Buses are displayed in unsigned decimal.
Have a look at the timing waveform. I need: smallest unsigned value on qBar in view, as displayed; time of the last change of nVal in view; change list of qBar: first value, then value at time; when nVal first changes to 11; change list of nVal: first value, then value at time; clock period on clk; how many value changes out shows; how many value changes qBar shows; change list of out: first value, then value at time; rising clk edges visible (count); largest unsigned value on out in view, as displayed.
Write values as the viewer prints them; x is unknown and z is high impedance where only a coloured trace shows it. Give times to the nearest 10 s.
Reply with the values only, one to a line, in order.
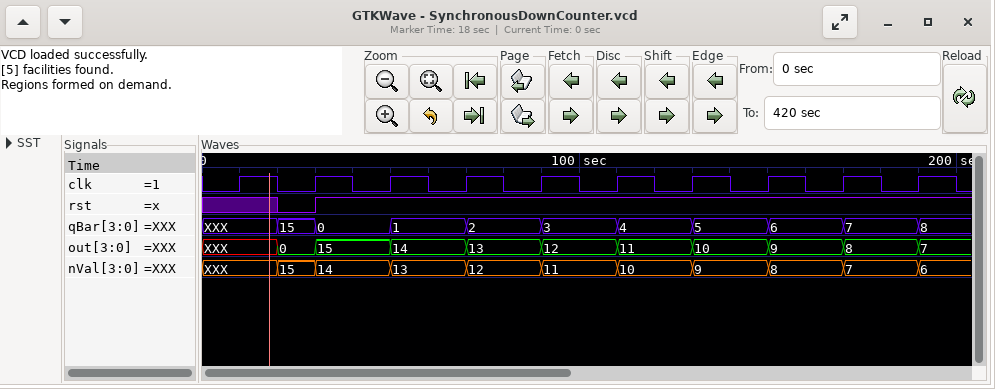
0
190 s
XXX, 15 at 20 s, 0 at 30 s, 1 at 50 s, 2 at 70 s, 3 at 90 s, 4 at 110 s, 5 at 130 s, 6 at 150 s, 7 at 170 s, 8 at 190 s
90 s
XXX, 15 at 20 s, 14 at 30 s, 13 at 50 s, 12 at 70 s, 11 at 90 s, 10 at 110 s, 9 at 130 s, 8 at 150 s, 7 at 170 s, 6 at 190 s
20 s
10
10
XXX, 0 at 20 s, 15 at 30 s, 14 at 50 s, 13 at 70 s, 12 at 90 s, 11 at 110 s, 10 at 130 s, 9 at 150 s, 8 at 170 s, 7 at 190 s
10
15
